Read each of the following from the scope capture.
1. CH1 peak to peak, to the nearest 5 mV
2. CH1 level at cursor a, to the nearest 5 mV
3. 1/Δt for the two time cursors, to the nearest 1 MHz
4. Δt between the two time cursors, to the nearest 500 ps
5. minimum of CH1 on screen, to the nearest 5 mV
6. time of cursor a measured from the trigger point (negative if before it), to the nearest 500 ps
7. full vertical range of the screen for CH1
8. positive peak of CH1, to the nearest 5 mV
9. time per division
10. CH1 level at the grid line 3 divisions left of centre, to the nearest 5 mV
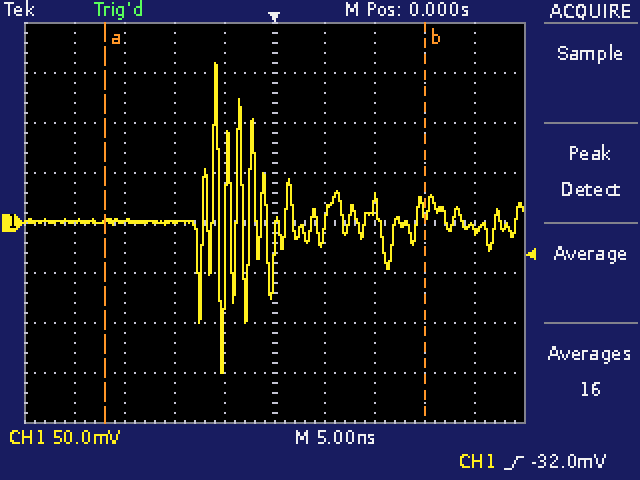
310 mV
0 mV
31 MHz
32.0 ns
-150 mV
-17.0 ns
400 mV
160 mV
5 ns
0 mV
